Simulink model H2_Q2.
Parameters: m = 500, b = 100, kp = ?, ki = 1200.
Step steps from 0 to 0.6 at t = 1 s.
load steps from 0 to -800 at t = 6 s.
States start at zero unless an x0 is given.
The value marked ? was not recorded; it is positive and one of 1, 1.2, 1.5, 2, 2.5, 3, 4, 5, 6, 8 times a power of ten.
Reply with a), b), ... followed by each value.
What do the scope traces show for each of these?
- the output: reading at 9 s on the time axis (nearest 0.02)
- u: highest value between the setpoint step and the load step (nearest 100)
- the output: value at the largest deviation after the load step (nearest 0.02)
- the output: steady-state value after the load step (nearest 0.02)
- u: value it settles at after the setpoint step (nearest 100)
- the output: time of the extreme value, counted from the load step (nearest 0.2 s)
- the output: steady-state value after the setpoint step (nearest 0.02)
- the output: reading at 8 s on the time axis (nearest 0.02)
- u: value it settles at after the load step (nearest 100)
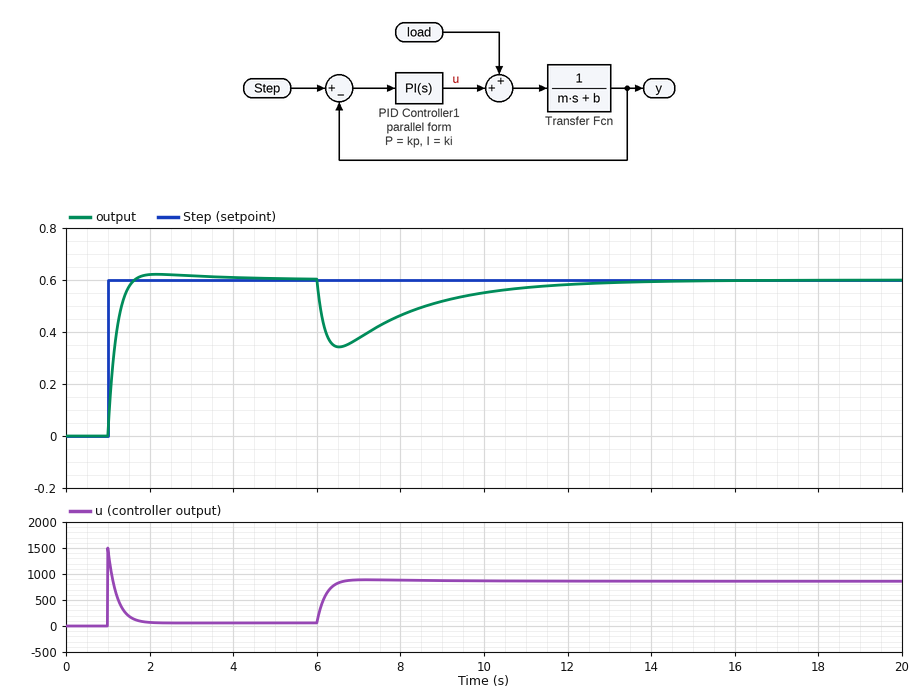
a) 0.52
b) 1500
c) 0.34
d) 0.60
e) 100
f) 0.6 s
g) 0.60
h) 0.46
i) 900
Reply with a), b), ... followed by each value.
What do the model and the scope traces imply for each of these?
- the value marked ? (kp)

a) 2500
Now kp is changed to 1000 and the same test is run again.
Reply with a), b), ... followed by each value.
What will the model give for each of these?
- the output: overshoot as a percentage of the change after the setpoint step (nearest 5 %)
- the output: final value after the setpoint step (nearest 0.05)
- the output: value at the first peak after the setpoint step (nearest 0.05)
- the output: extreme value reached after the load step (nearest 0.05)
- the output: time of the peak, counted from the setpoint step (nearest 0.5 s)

a) 15 %
b) 0.60
c) 0.70
d) 0.15
e) 1.5 s
